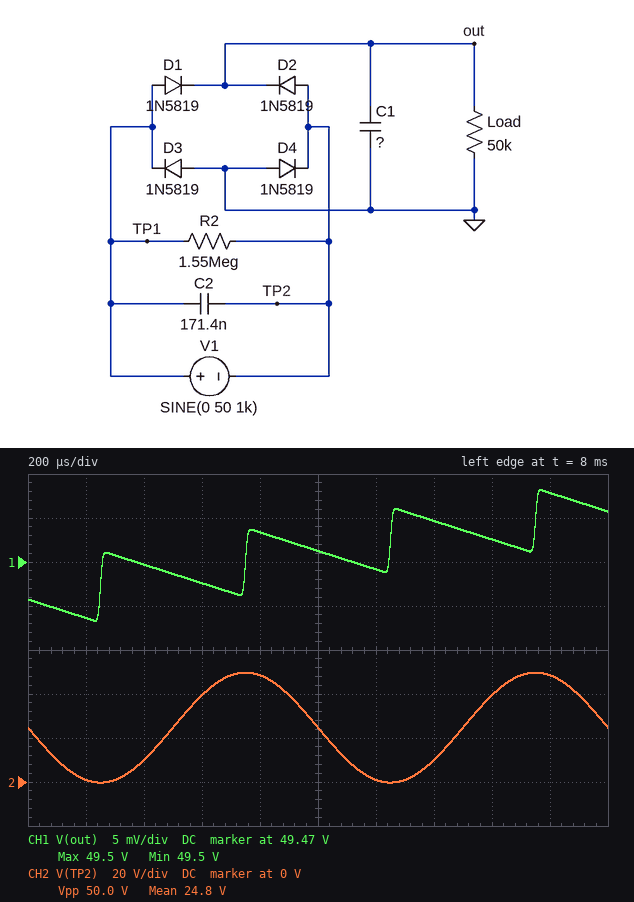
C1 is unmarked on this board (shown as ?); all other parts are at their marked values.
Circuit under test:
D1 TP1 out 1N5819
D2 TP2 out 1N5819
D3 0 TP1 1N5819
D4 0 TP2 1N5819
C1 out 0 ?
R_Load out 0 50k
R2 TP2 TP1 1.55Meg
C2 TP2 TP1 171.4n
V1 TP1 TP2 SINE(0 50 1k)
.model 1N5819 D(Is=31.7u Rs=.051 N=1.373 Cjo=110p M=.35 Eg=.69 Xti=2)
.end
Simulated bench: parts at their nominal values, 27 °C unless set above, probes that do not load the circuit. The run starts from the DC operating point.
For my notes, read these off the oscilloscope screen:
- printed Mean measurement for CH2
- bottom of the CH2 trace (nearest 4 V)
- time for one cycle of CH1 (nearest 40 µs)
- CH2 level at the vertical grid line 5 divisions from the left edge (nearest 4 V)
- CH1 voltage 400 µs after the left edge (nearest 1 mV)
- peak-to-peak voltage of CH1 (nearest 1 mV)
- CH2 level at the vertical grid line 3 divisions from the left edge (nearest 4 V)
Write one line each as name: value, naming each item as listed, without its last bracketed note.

printed Mean measurement for CH2: 24.8 V
bottom of the CH2 trace: 0 V
time for one cycle of CH1: 480 µs
CH2 level at the vertical grid line 5 divisions from the left edge: 24 V
CH1 voltage 400 µs after the left edge: 49.470 V
peak-to-peak voltage of CH1: 15 mV
CH2 level at the vertical grid line 3 divisions from the left edge: 40 V
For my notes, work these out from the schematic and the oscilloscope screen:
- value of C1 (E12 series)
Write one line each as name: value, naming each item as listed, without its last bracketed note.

value of C1: 100 µF
